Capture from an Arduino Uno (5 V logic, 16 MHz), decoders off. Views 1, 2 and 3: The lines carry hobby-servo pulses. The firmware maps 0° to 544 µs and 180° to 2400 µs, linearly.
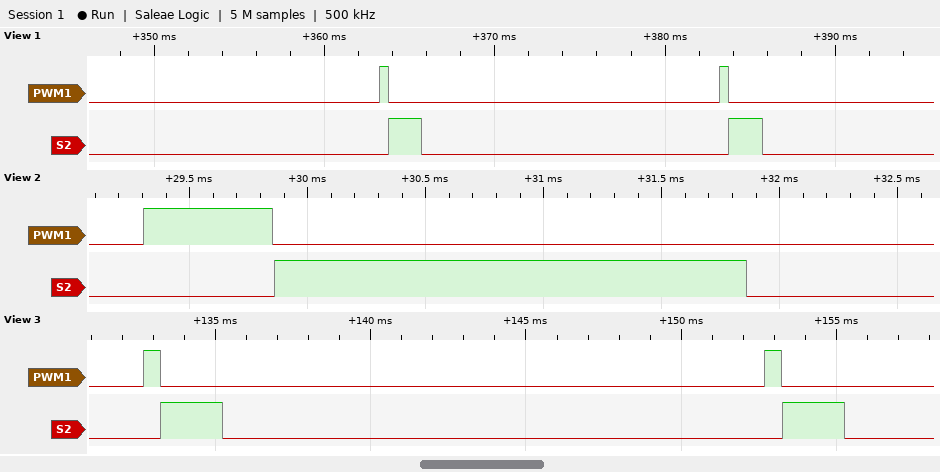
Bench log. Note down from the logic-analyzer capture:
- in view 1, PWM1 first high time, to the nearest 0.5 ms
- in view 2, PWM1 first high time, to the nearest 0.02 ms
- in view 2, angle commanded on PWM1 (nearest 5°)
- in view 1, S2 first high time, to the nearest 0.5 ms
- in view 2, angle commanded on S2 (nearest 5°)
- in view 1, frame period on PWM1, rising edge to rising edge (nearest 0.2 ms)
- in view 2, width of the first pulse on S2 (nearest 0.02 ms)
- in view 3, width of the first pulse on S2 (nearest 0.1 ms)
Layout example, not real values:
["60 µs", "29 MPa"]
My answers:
["0.5 ms", "0.54 ms", "0°", "2.0 ms", "140°", "20.0 ms", "2.00 ms", "2.0 ms"]
